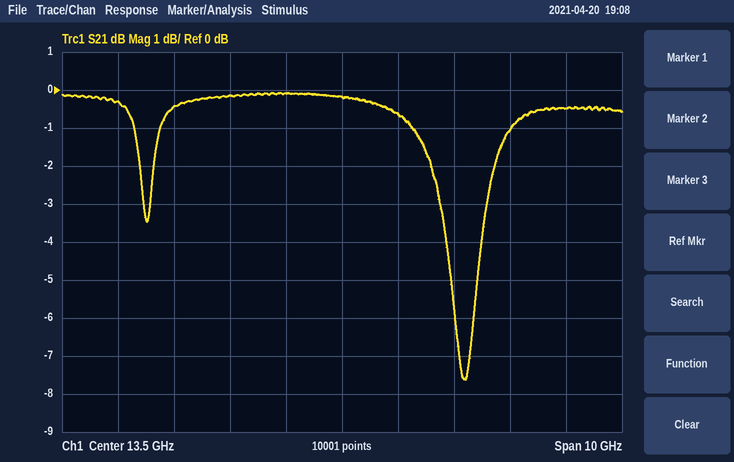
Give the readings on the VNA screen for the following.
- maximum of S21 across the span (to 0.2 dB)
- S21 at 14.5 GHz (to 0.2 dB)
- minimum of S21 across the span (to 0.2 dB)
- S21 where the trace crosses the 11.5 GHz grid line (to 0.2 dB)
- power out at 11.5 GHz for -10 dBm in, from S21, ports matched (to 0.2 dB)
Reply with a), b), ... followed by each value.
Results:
a) 0.0 dB
b) -0.6 dB
c) -7.6 dB
d) -0.2 dB
e) -10.2 dBm
